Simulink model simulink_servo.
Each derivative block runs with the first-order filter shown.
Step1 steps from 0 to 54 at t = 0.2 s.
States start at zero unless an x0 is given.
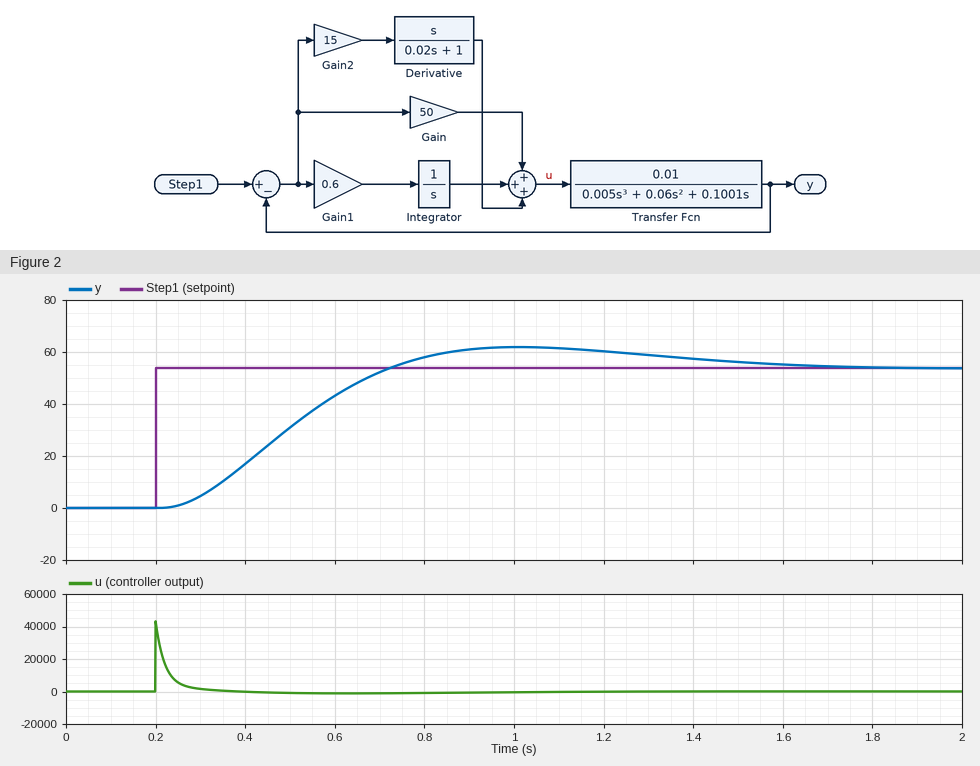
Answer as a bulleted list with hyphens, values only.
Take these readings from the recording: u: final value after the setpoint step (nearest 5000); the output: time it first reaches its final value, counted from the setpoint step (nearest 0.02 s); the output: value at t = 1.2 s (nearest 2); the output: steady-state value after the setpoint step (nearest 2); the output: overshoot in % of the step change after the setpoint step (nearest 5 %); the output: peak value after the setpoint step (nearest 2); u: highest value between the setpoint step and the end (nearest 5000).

- 0
- 0.52 s
- 60
- 54
- 15 %
- 62
- 45000
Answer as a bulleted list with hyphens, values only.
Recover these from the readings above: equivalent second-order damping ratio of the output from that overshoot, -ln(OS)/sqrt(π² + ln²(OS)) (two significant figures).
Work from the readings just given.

- 0.52
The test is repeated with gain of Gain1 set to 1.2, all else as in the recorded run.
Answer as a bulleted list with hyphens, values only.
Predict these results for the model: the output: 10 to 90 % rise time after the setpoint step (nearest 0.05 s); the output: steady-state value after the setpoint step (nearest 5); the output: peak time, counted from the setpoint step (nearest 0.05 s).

- 0.35 s
- 55
- 0.80 s
